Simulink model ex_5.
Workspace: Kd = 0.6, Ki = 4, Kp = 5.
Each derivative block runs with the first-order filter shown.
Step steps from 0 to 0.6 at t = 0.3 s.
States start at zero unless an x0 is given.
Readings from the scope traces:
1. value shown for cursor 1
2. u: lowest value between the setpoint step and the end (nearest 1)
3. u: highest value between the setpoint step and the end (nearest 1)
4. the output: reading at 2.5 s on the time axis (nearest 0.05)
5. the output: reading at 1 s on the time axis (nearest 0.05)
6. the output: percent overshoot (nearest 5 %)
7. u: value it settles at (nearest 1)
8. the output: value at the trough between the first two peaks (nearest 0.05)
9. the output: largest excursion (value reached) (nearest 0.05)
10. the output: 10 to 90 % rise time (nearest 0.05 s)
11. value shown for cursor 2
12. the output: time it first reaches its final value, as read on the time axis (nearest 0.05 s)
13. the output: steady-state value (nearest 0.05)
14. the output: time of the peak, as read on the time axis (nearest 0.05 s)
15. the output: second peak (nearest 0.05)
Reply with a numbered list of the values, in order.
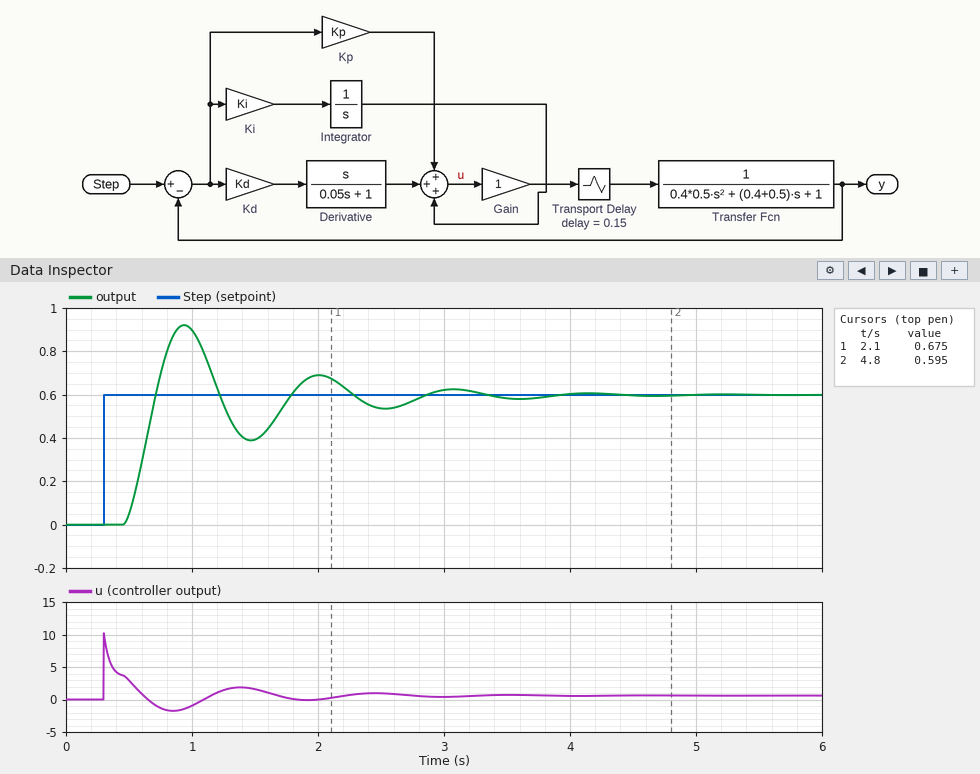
1. 0.675
2. -2
3. 10
4. 0.55
5. 0.90
6. 55 %
7. 1
8. 0.40
9. 0.90
10. 0.20 s
11. 0.595
12. 0.70 s
13. 0.60
14. 0.95 s
15. 0.70
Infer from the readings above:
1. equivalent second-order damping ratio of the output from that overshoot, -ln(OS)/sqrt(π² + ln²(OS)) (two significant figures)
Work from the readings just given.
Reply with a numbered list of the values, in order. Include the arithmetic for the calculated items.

1. ln(0.55) = -0.598; 0.598 / sqrt(9.870 + 0.357) = 0.19
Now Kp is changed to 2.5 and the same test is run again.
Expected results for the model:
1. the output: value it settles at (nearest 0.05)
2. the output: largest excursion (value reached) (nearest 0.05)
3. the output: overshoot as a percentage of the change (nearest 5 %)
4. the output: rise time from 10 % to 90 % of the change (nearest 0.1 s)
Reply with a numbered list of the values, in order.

1. 0.60
2. 0.70
3. 15 %
4. 0.3 s
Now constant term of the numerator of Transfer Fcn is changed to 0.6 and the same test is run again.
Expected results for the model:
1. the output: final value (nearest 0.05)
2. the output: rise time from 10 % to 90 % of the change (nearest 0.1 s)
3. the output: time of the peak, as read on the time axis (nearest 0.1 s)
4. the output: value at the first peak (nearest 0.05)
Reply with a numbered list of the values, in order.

1. 0.60
2. 0.3 s
3. 1.1 s
4. 0.70
